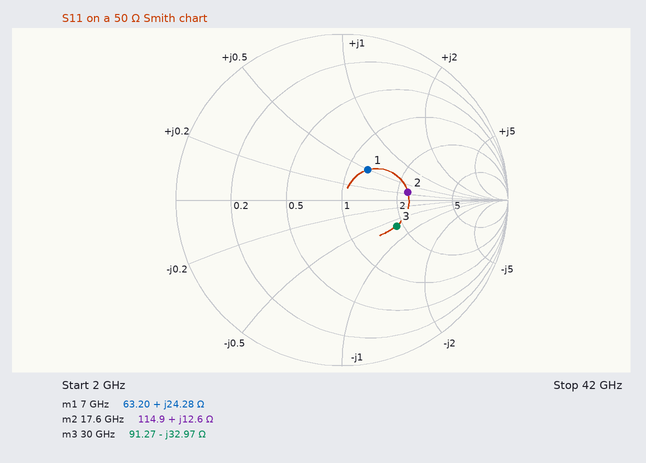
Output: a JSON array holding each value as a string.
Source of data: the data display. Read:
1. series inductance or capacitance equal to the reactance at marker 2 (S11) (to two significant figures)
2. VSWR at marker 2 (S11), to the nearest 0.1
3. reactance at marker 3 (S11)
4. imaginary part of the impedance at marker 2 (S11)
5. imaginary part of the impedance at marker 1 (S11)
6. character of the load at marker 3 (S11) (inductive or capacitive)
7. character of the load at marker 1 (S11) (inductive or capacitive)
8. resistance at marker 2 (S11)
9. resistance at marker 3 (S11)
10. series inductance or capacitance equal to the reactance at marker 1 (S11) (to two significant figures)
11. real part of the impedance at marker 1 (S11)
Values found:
["110 pH", "2.3", "-32.97 Ω", "+12.6 Ω", "+24.28 Ω", "capacitive", "inductive", "114.9 Ω", "91.27 Ω", "550 pH", "63.20 Ω"]
